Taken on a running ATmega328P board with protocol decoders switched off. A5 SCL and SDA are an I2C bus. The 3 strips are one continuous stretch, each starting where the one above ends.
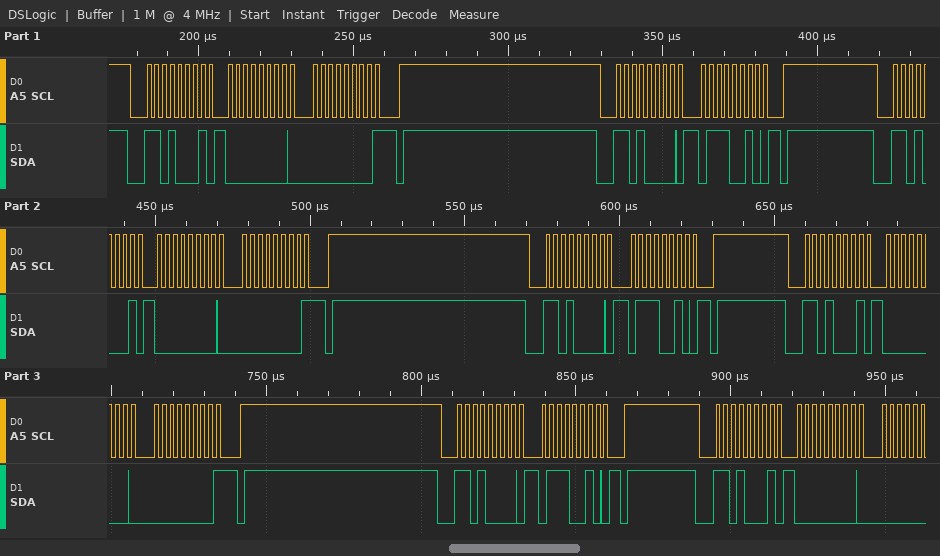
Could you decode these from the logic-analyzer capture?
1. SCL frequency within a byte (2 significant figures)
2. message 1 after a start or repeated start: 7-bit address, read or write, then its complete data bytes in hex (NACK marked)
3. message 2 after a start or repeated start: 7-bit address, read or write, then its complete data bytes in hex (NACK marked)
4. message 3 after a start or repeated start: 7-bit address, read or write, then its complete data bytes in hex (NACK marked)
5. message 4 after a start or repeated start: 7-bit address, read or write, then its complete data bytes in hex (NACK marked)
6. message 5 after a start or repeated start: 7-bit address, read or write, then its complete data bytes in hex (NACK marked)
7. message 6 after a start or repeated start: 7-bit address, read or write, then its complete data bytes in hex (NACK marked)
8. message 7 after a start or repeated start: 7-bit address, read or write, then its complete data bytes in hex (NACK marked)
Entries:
400 kHz
0x68 read: 00 00 NACK
0x68 write: 72
0x68 read: 00 00 NACK
0x68 write: 72
0x68 read: 00 00 NACK
0x68 write: 72
0x68 read: 00
